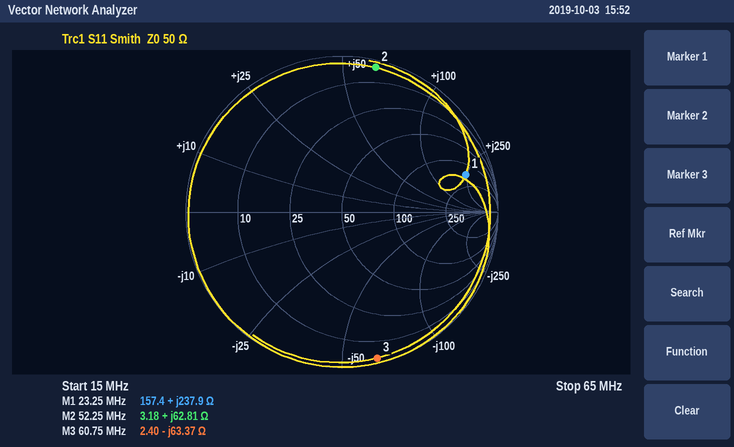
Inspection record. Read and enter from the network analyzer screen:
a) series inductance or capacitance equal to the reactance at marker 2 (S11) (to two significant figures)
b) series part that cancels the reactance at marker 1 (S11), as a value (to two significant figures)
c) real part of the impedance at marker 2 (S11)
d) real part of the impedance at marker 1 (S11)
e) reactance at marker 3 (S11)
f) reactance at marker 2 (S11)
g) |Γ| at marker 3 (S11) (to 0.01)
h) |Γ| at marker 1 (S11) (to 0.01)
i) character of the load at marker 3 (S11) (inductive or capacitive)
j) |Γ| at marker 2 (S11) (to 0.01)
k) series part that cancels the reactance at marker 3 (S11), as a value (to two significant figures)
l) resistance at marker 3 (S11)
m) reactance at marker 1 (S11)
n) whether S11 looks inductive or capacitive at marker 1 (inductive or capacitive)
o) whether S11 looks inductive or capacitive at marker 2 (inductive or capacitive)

190 nH
29 pF
3.18 Ω
157.4 Ω
-63.37 Ω
+62.81 Ω
0.96
0.83
capacitive
0.95
170 nH
2.40 Ω
+237.9 Ω
inductive
inductive
